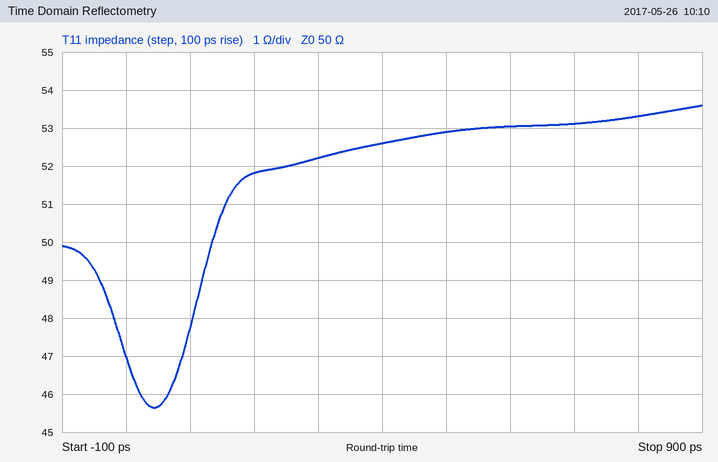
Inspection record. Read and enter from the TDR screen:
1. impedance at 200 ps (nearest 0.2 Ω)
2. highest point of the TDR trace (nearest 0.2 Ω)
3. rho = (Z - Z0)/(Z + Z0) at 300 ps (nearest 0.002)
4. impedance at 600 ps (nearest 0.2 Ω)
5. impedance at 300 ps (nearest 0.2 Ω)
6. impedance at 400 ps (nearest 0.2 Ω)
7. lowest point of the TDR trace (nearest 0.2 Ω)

51.8 Ω
53.6 Ω
+0.022
53.0 Ω
52.2 Ω
52.6 Ω
45.6 Ω
